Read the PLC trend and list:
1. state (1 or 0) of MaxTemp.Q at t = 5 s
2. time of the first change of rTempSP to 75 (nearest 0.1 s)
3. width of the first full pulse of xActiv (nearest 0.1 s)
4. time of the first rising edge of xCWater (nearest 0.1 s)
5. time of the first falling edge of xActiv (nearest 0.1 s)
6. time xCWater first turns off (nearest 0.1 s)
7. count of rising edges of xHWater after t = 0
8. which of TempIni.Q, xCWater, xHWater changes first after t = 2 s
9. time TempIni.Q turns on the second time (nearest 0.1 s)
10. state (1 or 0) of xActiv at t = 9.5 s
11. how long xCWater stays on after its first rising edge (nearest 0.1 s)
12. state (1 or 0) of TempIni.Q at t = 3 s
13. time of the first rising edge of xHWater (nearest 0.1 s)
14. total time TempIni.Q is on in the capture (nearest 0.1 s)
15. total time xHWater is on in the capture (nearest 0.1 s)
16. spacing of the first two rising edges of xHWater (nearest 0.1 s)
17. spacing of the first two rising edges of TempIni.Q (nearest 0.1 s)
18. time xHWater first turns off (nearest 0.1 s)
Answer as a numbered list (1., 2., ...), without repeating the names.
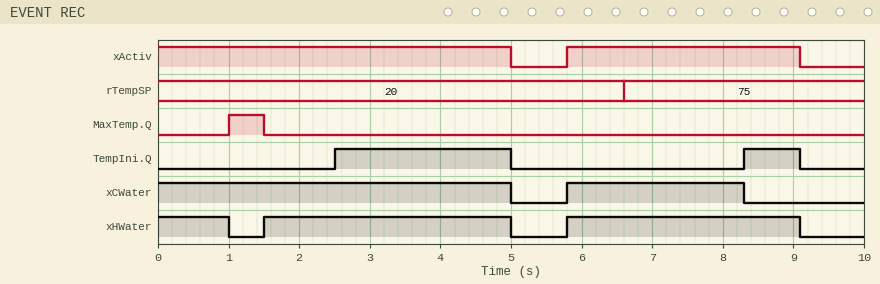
1. 0
2. 6.6 s
3. 3.3 s
4. 5.8 s
5. 5.0 s
6. 5.0 s
7. 2
8. TempIni.Q
9. 8.3 s
10. 0
11. 2.5 s
12. 1
13. 1.5 s
14. 3.3 s
15. 7.8 s
16. 4.3 s
17. 5.8 s
18. 1.0 s
